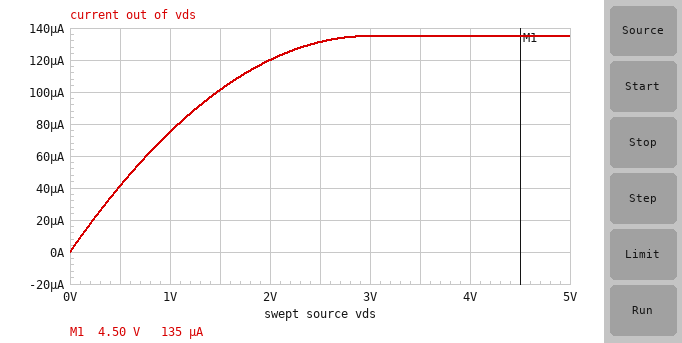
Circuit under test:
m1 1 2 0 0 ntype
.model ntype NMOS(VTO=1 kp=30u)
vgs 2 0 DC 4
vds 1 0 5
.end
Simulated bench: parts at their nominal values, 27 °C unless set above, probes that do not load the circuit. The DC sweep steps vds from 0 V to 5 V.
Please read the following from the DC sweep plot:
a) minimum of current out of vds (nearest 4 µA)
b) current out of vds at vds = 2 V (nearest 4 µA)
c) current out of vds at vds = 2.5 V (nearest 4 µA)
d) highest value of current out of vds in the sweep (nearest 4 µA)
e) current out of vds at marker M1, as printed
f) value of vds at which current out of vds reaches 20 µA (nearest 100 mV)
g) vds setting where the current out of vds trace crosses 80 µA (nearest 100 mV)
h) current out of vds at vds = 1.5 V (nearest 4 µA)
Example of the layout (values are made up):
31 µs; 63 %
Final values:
0 A; 120 µA; 132 µA; 136 µA; 135 µA; 200 mV; 1.1 V; 100 µA
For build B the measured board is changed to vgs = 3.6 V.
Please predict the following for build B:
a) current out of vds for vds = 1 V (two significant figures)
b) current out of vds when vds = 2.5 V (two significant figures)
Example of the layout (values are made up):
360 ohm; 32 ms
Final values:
63 µA; 100 µA
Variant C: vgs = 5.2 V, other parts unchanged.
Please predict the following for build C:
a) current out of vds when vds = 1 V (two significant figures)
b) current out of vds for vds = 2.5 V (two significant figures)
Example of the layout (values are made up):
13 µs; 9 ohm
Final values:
110 µA; 220 µA
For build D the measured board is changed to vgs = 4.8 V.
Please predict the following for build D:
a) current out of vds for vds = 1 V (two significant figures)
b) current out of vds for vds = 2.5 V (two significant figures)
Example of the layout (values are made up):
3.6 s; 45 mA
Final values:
99 µA; 190 µA
